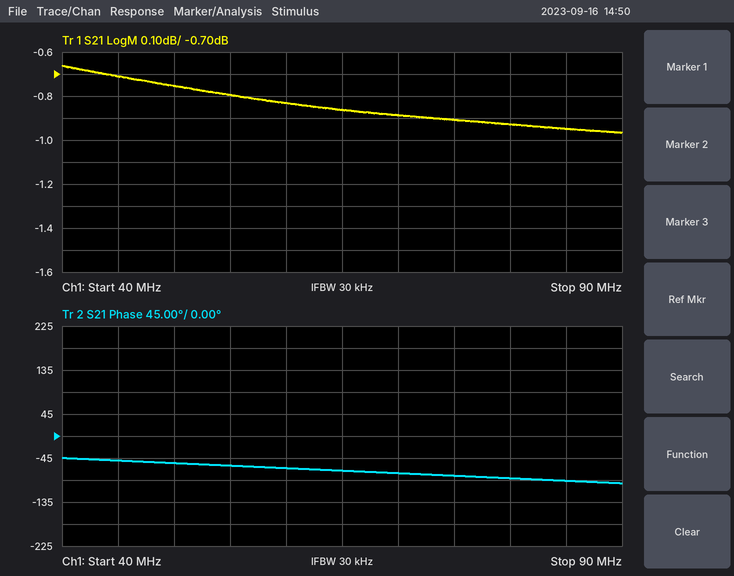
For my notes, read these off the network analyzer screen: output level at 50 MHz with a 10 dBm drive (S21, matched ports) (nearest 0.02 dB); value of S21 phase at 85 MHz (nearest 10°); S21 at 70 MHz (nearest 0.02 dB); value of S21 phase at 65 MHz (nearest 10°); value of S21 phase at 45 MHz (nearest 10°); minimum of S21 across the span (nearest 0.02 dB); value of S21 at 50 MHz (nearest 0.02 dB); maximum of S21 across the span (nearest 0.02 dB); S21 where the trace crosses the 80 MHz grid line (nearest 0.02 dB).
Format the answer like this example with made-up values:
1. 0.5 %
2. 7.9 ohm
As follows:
1. 9.24 dBm
2. -90°
3. -0.88 dB
4. -70°
5. -50°
6. -0.96 dB
7. -0.76 dB
8. -0.66 dB
9. -0.92 dB
